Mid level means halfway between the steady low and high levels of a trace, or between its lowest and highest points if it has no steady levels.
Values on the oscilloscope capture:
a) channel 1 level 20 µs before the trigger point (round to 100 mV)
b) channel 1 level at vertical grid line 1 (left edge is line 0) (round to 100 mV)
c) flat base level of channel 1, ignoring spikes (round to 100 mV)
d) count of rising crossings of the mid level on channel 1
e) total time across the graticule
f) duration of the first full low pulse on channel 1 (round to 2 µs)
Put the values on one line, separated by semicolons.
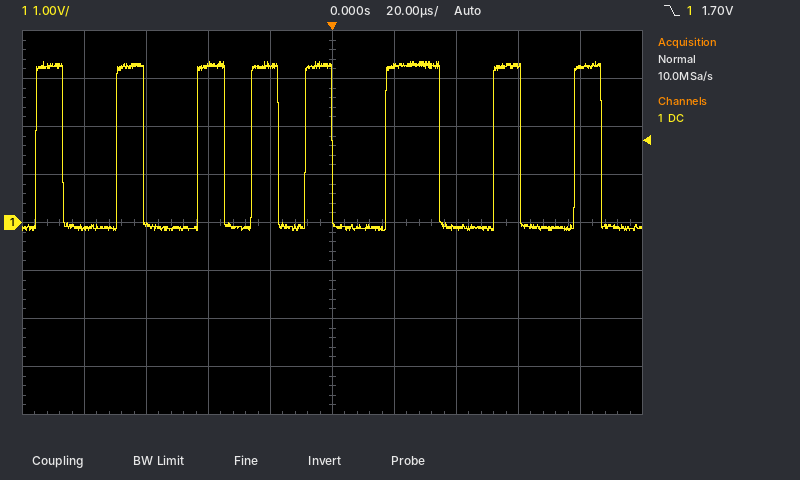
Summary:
3.3 V; -100 mV; -100 mV; 8; 200 µs; 18 µs
